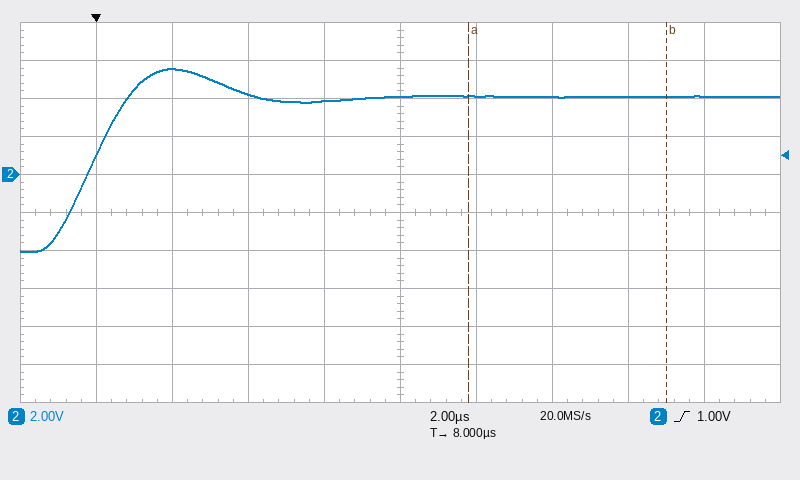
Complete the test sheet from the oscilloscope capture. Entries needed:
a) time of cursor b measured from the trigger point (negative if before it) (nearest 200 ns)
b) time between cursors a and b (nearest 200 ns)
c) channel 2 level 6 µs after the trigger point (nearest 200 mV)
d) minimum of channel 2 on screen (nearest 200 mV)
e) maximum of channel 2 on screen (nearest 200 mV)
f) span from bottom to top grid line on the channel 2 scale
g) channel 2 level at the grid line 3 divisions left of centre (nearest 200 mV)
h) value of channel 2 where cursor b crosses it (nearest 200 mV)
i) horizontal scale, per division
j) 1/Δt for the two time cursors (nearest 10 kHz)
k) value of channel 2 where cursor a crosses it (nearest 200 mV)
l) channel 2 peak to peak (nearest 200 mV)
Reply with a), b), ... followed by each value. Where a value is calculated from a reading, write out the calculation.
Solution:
a) +15.0 µs
b) 5.2 µs
c) 3.8 V
d) -4.0 V
e) 5.6 V
f) 20 V
g) 5.6 V
h) 4.2 V
i) 2 µs
j) 1 / 5.2 µs ≈ 190 kHz
k) 4.2 V
l) 5.6 V − (-4.0 V) = 9.6 V
